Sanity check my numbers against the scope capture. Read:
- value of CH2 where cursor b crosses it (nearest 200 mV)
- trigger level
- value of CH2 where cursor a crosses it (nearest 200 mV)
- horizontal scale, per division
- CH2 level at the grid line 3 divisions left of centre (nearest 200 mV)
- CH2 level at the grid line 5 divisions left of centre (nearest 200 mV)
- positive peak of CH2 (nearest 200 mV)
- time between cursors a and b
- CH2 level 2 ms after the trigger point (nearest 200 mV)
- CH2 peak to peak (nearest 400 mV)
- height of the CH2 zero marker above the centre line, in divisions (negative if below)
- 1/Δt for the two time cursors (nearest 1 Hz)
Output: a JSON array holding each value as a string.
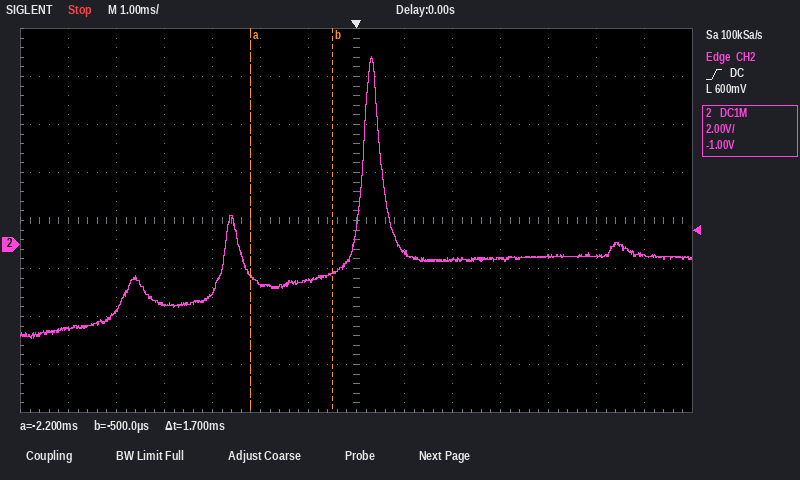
["-1.2 V", "600 mV", "-1.2 V", "1 ms", "-2.0 V", "-2.8 V", "7.8 V", "1.7 ms", "-600 mV", "11.6 V", "-0.5 div", "588 Hz"]
